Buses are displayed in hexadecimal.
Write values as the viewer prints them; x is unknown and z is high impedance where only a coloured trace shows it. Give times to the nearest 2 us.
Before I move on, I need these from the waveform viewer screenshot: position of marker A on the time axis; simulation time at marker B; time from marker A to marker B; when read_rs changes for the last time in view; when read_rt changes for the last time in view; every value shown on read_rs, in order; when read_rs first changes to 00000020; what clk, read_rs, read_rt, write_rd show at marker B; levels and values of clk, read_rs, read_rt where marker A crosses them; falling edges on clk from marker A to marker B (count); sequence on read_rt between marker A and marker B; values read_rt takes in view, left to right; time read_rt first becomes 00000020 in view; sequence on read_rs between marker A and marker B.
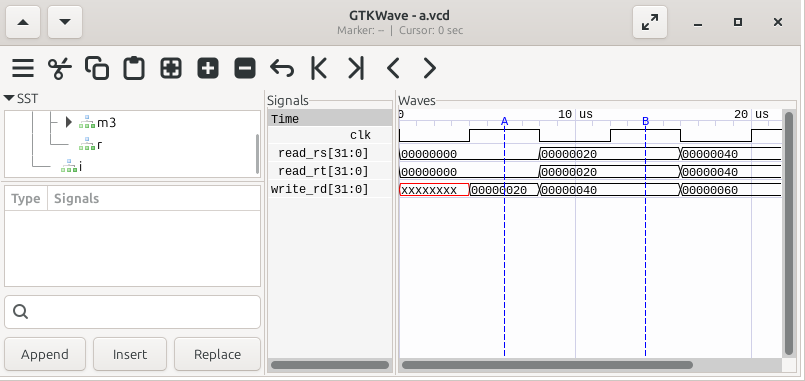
6 us
14 us
8 us
16 us
16 us
00000000, 00000020, 00000040
8 us
clk=1, read_rs=00000020, read_rt=00000020, write_rd=00000040
clk=1, read_rs=00000000, read_rt=00000000
1
00000000, 00000020
00000000, 00000020, 00000040
8 us
00000000, 00000020
